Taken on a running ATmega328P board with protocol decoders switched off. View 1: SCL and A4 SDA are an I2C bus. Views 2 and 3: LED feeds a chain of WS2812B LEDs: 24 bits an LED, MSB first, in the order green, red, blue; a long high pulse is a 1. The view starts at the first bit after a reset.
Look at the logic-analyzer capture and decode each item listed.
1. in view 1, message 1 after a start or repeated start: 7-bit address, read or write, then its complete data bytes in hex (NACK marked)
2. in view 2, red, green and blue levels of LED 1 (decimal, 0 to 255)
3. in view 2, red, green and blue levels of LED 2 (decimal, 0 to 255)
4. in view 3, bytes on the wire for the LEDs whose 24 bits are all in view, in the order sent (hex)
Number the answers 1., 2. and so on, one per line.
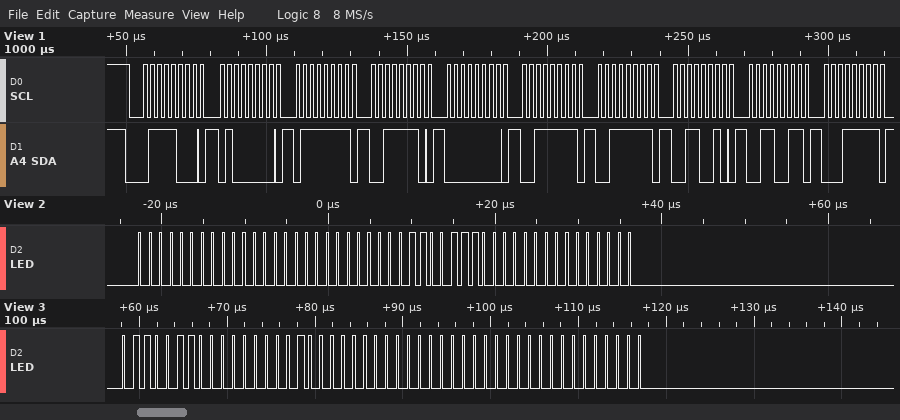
1. 0x3C write: 40 7F 3E 00 3F 3F 32 33 1F
2. 0, 0, 0
3. 128, 51, 0
4. 66 00 80 00 00 00
